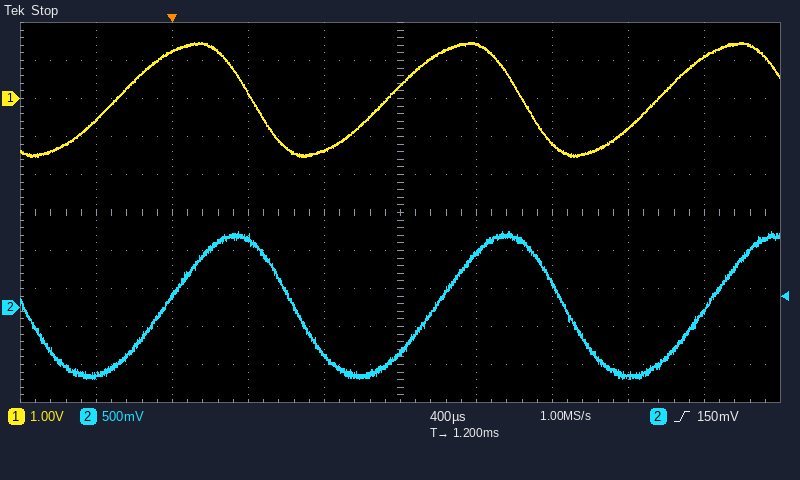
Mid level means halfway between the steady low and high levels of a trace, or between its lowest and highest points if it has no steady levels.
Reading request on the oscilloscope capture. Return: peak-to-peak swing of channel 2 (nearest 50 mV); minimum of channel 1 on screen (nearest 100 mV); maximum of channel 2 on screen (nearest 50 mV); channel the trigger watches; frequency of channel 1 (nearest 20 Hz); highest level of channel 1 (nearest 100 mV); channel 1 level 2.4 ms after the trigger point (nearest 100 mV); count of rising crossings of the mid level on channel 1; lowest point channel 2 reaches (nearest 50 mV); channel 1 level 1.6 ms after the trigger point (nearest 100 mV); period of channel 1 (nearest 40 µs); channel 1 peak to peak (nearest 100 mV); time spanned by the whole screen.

1.95 V
-1.5 V
1.00 V
channel 2
700 Hz
1.5 V
-800 mV
3
-950 mV
1.4 V
1.44 ms
3.0 V
4 ms
